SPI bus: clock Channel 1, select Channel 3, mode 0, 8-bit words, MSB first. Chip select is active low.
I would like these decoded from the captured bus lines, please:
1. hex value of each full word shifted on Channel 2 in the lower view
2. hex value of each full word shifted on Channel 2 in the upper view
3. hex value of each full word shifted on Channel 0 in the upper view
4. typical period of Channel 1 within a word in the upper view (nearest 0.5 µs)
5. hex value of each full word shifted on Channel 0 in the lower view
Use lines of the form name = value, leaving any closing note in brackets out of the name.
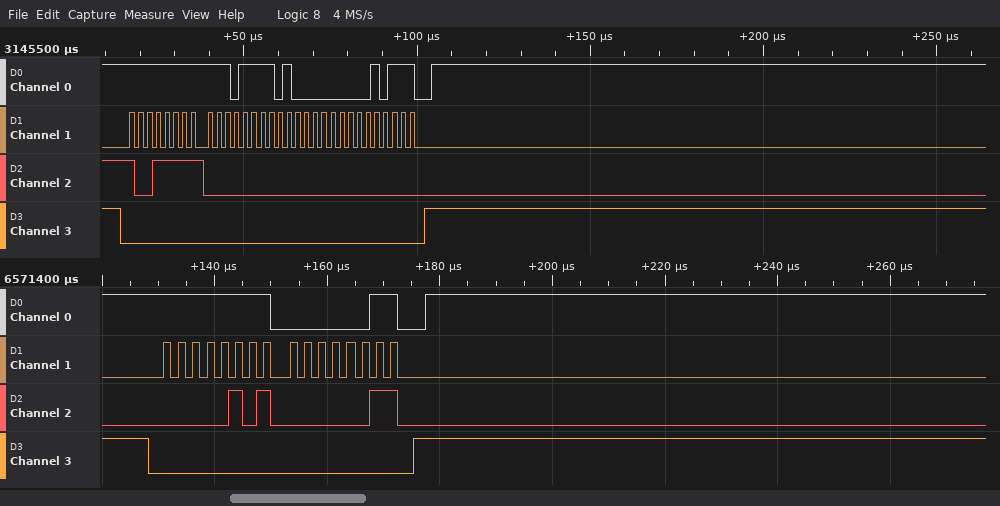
hex value of each full word shifted on Channel 2 in the lower view = 05, 03
hex value of each full word shifted on Channel 2 in the upper view = 9F, 00, 00, 00
hex value of each full word shifted on Channel 0 in the upper view = FF, EF, 40, 17
typical period of Channel 1 within a word in the upper view = 2.5 µs
hex value of each full word shifted on Channel 0 in the lower view = FF, 03
